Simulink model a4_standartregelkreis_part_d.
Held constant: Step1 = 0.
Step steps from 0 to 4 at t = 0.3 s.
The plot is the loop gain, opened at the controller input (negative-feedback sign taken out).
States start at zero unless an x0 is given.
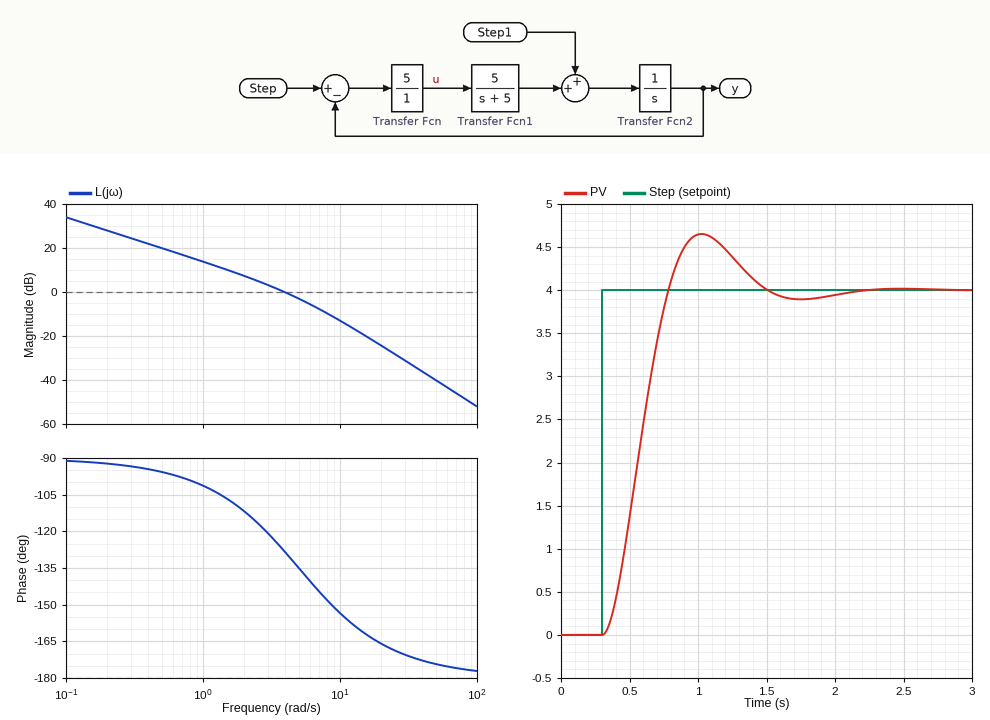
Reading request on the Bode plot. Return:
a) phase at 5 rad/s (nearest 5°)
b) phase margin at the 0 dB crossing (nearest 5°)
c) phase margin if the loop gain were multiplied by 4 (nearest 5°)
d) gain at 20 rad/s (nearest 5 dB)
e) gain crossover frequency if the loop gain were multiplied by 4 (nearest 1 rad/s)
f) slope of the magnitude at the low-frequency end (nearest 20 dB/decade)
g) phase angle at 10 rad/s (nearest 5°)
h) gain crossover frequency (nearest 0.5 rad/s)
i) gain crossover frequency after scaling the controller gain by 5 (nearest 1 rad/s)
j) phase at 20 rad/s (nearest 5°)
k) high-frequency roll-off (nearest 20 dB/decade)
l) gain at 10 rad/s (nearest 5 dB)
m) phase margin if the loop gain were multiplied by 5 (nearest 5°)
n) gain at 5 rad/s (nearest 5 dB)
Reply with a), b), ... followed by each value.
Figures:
a) -135°
b) 50°
c) 30°
d) -25 dB
e) 9 rad/s
f) -20 dB/decade
g) -155°
h) 4.0 rad/s
i) 11 rad/s
j) -165°
k) -40 dB/decade
l) -15 dB
m) 25°
n) -5 dB
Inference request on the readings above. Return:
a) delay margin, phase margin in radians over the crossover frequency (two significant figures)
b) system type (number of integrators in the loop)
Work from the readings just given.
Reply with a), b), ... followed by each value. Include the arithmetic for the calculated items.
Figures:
a) 50 × π / 180 / 4 = 0.22 s
b) 1
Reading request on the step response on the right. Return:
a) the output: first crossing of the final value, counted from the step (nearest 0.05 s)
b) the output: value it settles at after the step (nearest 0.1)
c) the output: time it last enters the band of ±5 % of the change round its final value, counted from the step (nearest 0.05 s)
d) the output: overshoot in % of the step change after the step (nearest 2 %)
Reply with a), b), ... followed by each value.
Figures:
a) 0.50 s
b) 4.0
c) 1.05 s
d) 16 %
